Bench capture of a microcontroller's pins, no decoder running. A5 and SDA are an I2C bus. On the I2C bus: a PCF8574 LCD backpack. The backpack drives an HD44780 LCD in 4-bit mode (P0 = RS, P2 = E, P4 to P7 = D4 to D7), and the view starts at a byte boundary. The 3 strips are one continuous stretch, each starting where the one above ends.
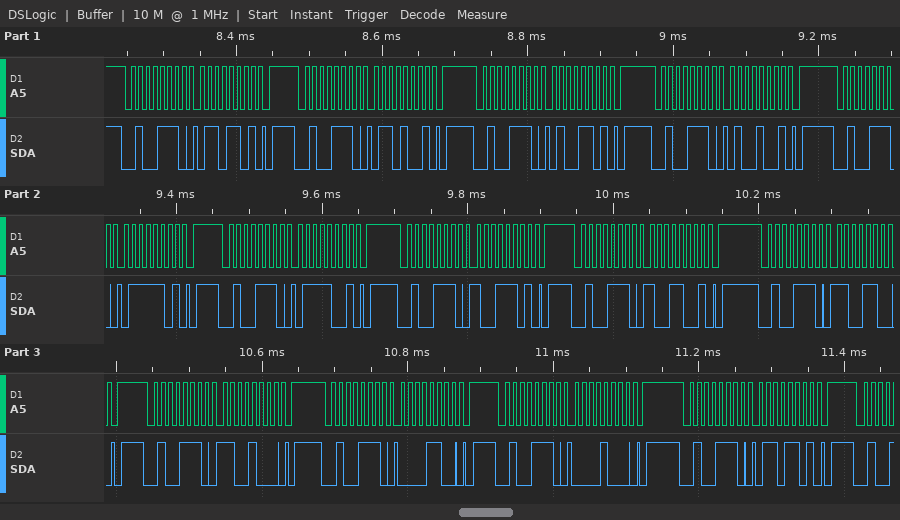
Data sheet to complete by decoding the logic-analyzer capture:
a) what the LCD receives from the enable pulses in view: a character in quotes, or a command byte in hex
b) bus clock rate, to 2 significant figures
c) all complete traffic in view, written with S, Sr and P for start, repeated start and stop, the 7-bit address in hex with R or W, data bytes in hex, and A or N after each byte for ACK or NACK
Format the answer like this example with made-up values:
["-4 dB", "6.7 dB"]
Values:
["'d' 'y' 0xC0", "100 kHz", "S 27W A 6D A P S 27W A 69 A P S 27W A 4D A P S 27W A 49 A P S 27W A 7D A P S 27W A 79 A P S 27W A 9D A P S 27W A 99 A P S 27W A CC A P S 27W A C8 A P S 27W A 0C A P S 27W A 08 A P S 27W A 6D A P"]
